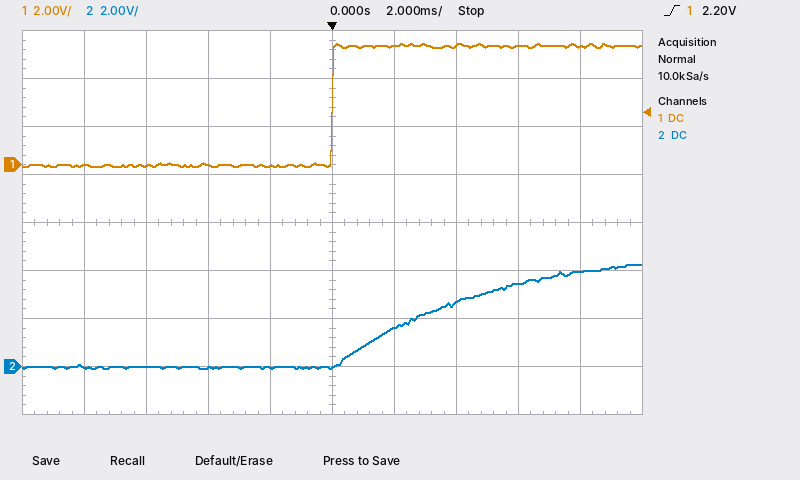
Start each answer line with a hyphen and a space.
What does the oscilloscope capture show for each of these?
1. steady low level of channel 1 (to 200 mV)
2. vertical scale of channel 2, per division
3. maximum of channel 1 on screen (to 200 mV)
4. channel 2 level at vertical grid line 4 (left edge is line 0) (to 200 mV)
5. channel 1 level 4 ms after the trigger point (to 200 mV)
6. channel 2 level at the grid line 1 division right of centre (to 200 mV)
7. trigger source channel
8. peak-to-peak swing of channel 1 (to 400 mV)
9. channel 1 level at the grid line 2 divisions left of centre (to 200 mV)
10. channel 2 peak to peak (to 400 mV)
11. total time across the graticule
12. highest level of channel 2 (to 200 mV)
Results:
- 0.0 V
- 2 V
- 5.0 V
- 0.0 V
- 5.0 V
- 1.6 V
- channel 1
- 5.2 V
- 0.0 V
- 4.4 V
- 20 ms
- 4.2 V
